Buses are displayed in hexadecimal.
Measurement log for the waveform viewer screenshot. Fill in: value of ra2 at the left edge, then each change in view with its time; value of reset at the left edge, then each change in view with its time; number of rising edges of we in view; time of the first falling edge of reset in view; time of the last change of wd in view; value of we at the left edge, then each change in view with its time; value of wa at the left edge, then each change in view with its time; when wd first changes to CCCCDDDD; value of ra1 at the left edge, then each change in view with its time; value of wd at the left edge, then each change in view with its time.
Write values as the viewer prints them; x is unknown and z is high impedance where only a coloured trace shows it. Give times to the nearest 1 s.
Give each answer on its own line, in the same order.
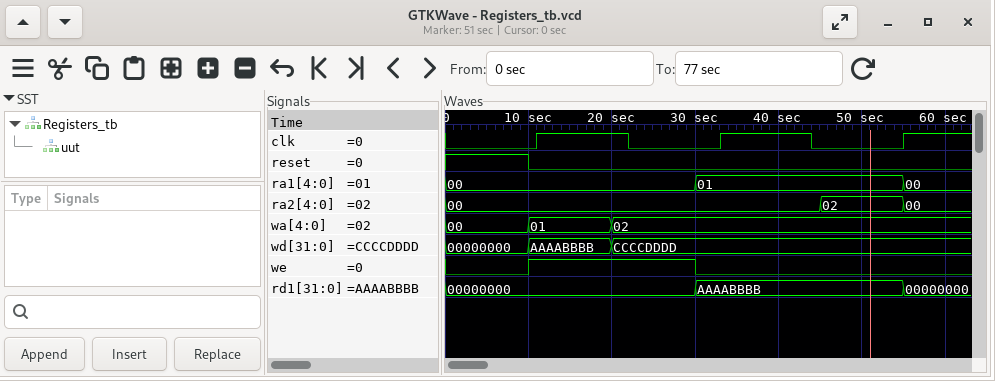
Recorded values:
00, 02 at 45 s, 00 at 55 s
1, 0 at 10 s
1
10 s
20 s
0, 1 at 10 s, 0 at 30 s
00, 01 at 10 s, 02 at 20 s
20 s
00, 01 at 30 s, 00 at 55 s
00000000, AAAABBBB at 10 s, CCCCDDDD at 20 s
